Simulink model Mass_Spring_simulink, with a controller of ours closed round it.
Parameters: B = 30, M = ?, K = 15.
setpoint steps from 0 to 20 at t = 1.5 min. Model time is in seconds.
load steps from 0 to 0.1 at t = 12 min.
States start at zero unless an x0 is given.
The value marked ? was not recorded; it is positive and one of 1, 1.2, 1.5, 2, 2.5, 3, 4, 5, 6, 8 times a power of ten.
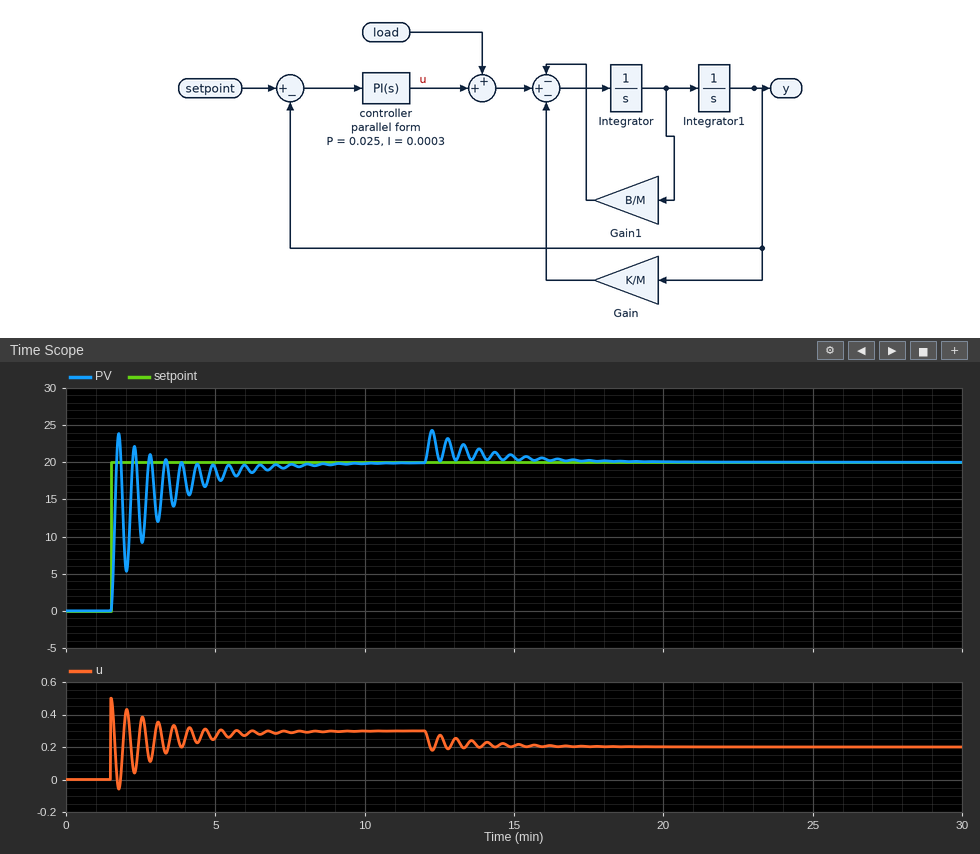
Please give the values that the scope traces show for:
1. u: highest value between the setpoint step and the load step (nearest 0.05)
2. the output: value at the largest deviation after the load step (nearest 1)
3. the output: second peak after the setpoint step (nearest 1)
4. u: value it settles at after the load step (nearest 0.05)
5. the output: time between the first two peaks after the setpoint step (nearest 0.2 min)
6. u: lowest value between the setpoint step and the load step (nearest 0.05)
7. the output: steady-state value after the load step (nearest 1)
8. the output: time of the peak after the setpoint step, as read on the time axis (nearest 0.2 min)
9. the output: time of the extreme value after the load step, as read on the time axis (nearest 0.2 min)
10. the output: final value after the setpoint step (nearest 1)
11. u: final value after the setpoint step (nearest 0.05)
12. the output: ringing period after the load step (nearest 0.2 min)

0.50
24
22
0.20
0.6 min
-0.05
20
1.8 min
12.2 min
20
0.30
0.6 min
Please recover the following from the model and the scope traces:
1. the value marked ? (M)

1000
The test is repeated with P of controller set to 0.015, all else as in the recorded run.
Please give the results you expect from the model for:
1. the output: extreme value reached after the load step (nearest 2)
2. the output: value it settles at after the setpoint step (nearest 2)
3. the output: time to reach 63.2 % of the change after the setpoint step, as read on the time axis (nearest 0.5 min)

26
20
1.5 min
